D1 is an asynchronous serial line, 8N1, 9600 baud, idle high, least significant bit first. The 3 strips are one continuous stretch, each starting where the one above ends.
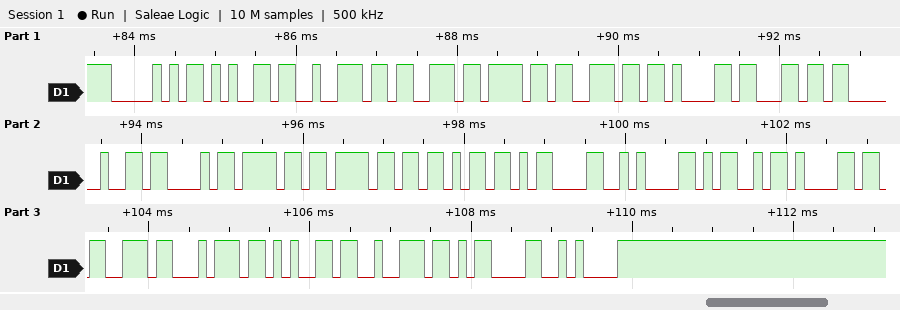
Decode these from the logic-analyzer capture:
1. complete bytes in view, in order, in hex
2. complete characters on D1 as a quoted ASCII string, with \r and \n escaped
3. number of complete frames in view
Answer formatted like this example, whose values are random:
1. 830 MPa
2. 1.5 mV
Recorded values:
1. 50 65 72 73 6F 6E 61 6C 20 43 6F 6F 6B 0D 0A 4D 61 73 74 65 72 0D 0A
2. "Personal Cook\r\nMaster\r\n"
3. 23
